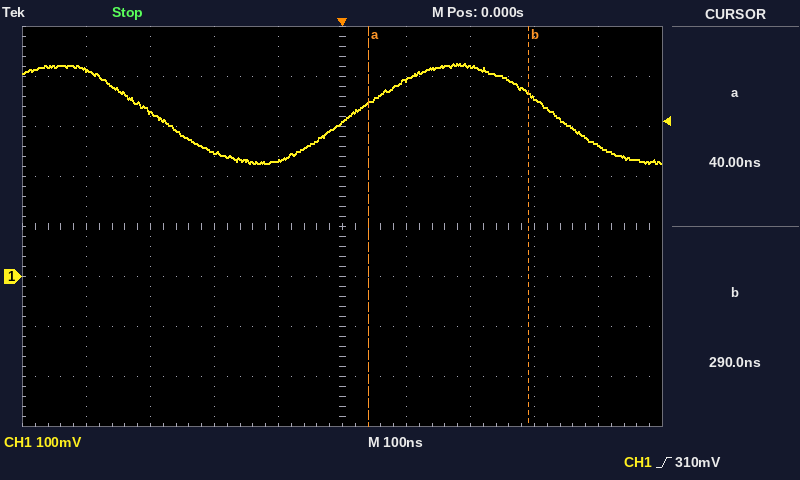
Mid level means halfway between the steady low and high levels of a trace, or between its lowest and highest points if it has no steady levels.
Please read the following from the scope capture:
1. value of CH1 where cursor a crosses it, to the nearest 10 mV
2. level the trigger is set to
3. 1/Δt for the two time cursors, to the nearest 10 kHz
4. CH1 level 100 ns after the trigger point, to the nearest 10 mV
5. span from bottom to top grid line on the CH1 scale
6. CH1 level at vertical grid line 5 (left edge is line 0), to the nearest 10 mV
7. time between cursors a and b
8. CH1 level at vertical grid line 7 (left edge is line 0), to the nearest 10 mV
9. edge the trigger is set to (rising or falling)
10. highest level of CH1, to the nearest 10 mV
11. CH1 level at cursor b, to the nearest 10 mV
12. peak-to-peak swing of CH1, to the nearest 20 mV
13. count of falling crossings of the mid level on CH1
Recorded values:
350 mV
310 mV
4.00 MHz
390 mV
800 mV
310 mV
250 ns
420 mV
rising
430 mV
370 mV
200 mV
2
